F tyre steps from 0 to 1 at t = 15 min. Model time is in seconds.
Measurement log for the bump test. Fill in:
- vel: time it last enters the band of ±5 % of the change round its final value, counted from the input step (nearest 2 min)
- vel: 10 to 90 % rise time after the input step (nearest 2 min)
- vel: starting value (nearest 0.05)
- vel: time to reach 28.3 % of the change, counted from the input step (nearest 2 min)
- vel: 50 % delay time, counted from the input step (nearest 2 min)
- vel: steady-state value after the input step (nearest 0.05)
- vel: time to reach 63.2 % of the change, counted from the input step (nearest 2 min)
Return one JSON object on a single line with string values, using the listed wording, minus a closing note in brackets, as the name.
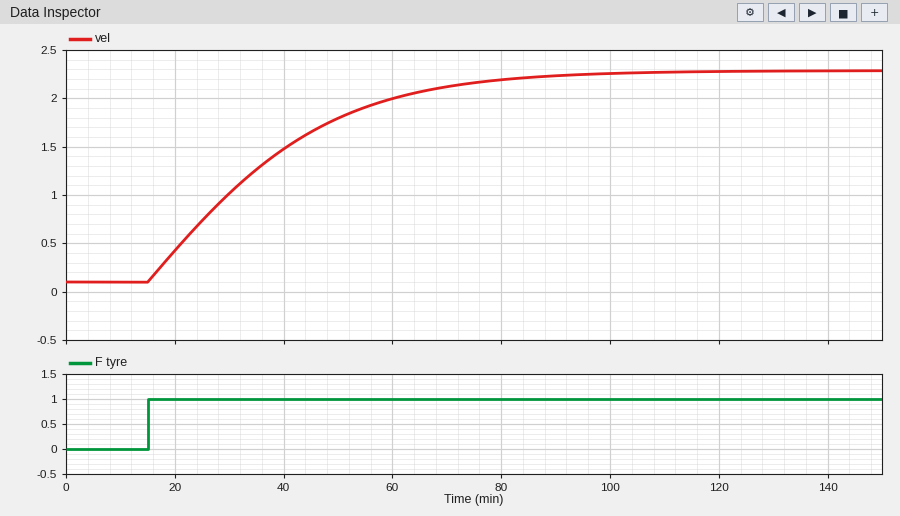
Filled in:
{"vel: time it last enters the band of ±5 % of the change round its final value, counted from the input step": "62 min", "vel: 10 to 90 % rise time after the input step": "46 min", "vel: starting value": "0.10", "vel: time to reach 28.3 % of the change, counted from the input step": "10 min", "vel: 50 % delay time, counted from the input step": "18 min", "vel: steady-state value after the input step": "2.30", "vel: time to reach 63.2 % of the change, counted from the input step": "26 min"}
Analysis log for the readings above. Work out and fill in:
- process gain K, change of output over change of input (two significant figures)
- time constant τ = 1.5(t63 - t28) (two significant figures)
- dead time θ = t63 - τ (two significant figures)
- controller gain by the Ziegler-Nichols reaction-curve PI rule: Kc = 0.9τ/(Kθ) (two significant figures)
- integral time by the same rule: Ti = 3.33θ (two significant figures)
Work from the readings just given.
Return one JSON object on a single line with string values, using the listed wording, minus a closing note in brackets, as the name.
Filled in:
{"process gain K, change of output over change of input": "2.2", "time constant τ = 1.5(t63 - t28)": "24 min", "dead time θ = t63 - τ": "2.0 min", "controller gain by the Ziegler-Nichols reaction-curve PI rule: Kc = 0.9τ/(Kθ)": "4.9", "integral time by the same rule: Ti = 3.33θ": "6.7 min"}
